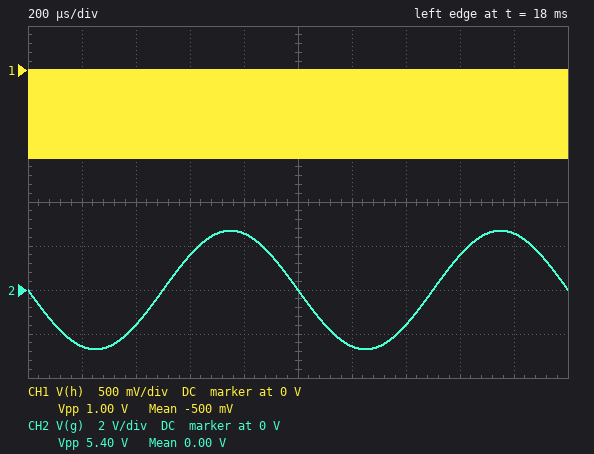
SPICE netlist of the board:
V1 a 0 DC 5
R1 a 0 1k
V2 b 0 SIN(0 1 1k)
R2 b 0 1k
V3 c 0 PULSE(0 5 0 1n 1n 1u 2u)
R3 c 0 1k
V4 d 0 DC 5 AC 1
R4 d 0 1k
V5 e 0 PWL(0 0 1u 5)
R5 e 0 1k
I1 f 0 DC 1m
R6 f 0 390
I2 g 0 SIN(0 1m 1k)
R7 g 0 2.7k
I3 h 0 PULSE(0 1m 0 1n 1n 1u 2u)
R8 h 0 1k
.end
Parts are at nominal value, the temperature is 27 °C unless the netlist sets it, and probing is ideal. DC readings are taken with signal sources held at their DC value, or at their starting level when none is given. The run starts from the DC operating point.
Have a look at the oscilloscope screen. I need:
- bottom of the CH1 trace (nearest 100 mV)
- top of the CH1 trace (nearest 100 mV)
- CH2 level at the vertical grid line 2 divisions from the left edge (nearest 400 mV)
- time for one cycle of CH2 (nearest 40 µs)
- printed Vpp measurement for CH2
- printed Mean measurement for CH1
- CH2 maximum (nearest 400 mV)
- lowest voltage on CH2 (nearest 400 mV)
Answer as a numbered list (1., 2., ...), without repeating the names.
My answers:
1. -1.0 V
2. 0 V
3. -1.6 V
4. 1.00 ms
5. 5.40 V
6. -500 mV
7. 2.8 V
8. -2.8 V
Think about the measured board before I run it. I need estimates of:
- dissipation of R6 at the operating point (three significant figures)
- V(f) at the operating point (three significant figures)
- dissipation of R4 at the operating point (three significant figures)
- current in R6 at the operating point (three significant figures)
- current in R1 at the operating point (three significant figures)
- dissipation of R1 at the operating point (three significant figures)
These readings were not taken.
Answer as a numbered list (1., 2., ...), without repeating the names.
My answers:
1. 390 µW
2. -390 mV
3. 25.0 mW
4. 1.00 mA
5. 5.00 mA
6. 25.0 mW
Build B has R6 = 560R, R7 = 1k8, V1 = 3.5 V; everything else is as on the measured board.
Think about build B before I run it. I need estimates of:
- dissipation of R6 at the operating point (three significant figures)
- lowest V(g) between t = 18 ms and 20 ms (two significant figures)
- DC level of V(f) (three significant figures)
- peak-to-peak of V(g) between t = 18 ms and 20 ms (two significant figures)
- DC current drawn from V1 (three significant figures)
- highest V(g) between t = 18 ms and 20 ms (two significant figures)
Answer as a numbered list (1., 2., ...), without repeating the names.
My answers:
1. 560 µW
2. -1.8 V
3. -560 mV
4. 3.6 V
5. 3.50 mA
6. 1.8 V
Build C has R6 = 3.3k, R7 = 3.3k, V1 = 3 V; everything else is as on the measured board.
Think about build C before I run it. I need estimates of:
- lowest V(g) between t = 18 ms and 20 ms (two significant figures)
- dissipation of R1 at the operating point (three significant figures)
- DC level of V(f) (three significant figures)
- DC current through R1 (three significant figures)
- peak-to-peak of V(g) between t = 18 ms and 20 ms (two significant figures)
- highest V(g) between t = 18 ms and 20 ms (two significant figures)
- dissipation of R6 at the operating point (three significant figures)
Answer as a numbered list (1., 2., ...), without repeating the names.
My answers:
1. -3.3 V
2. 9.00 mW
3. -3.30 V
4. 3.00 mA
5. 6.6 V
6. 3.3 V
7. 3.30 mW
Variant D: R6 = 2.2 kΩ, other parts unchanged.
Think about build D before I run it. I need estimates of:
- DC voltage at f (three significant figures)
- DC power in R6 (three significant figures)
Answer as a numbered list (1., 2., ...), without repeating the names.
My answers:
1. -2.20 V
2. 2.20 mW
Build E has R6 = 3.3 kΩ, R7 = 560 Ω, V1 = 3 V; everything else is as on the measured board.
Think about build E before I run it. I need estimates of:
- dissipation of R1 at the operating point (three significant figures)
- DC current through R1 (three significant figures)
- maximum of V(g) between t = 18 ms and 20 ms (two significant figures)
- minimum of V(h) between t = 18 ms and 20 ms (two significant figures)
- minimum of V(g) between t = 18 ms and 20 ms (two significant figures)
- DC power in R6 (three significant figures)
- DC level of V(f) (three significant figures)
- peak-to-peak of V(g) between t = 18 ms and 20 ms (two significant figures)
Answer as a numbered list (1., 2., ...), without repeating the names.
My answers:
1. 9.00 mW
2. 3.00 mA
3. 560 mV
4. -1.0 V
5. -560 mV
6. 3.30 mW
7. -3.30 V
8. 1.1 V
